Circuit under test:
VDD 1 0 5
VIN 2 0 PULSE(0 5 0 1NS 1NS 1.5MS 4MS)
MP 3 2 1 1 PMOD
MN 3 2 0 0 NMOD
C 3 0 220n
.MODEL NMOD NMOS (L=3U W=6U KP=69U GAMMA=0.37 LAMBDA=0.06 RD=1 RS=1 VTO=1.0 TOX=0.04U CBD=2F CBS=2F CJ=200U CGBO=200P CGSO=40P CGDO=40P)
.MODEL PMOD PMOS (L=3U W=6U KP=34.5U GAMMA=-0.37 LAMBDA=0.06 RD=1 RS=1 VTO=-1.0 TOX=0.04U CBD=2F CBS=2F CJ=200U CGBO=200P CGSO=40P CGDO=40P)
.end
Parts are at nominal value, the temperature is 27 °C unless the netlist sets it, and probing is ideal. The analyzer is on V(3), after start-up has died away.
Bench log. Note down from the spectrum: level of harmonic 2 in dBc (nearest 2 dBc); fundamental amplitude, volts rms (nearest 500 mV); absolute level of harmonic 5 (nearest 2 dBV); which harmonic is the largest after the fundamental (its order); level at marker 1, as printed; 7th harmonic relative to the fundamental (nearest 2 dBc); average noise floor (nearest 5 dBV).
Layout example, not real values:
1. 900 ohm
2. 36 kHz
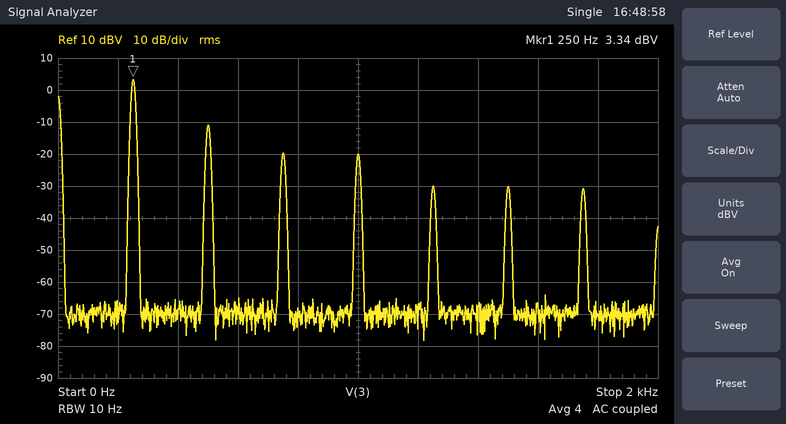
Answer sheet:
1. -14 dBc
2. 1.5 V
3. -30 dBV
4. 2
5. 3.34 dBV
6. -34 dBc
7. -70 dBV
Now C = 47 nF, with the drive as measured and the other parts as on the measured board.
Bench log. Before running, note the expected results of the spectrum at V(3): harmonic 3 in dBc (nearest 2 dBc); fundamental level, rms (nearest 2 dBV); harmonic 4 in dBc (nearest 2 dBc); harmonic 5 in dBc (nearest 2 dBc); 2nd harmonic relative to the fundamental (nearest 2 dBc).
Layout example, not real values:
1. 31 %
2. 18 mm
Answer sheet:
1. -16 dBc
2. 6 dBV
3. -14 dBc
4. -28 dBc
5. -10 dBc
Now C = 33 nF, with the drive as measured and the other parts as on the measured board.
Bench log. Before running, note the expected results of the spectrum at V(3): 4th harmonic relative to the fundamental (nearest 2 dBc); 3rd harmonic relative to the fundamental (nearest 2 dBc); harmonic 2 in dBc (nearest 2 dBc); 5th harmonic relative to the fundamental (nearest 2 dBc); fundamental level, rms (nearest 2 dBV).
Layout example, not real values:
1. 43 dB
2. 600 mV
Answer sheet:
1. -14 dBc
2. -16 dBc
3. -10 dBc
4. -28 dBc
5. 6 dBV
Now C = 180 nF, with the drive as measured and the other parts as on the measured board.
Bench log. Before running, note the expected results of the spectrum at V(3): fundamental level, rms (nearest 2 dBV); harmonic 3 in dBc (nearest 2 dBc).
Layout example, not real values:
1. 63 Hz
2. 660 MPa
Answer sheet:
1. 4 dBV
2. -22 dBc
